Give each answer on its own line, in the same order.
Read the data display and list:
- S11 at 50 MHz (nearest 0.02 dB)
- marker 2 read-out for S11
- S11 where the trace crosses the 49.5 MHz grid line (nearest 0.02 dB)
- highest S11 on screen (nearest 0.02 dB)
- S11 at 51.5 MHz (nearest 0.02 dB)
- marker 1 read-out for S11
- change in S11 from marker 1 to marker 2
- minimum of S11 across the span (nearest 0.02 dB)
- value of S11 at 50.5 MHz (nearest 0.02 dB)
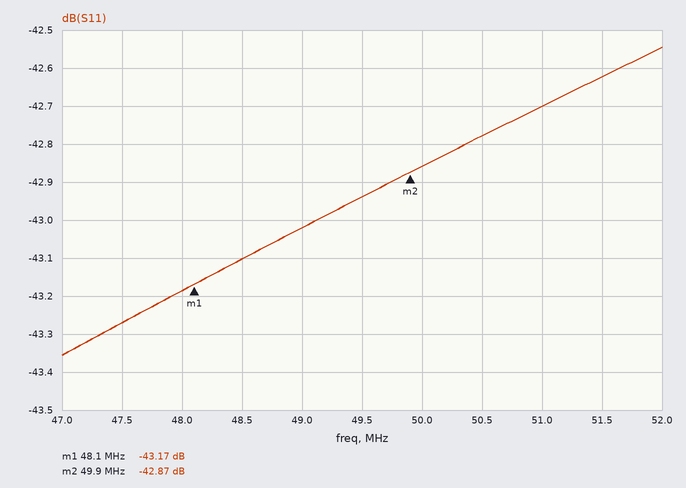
-42.86 dB
-42.87 dB
-42.94 dB
-42.54 dB
-42.62 dB
-43.17 dB
0.30 dB
-43.36 dB
-42.78 dB
